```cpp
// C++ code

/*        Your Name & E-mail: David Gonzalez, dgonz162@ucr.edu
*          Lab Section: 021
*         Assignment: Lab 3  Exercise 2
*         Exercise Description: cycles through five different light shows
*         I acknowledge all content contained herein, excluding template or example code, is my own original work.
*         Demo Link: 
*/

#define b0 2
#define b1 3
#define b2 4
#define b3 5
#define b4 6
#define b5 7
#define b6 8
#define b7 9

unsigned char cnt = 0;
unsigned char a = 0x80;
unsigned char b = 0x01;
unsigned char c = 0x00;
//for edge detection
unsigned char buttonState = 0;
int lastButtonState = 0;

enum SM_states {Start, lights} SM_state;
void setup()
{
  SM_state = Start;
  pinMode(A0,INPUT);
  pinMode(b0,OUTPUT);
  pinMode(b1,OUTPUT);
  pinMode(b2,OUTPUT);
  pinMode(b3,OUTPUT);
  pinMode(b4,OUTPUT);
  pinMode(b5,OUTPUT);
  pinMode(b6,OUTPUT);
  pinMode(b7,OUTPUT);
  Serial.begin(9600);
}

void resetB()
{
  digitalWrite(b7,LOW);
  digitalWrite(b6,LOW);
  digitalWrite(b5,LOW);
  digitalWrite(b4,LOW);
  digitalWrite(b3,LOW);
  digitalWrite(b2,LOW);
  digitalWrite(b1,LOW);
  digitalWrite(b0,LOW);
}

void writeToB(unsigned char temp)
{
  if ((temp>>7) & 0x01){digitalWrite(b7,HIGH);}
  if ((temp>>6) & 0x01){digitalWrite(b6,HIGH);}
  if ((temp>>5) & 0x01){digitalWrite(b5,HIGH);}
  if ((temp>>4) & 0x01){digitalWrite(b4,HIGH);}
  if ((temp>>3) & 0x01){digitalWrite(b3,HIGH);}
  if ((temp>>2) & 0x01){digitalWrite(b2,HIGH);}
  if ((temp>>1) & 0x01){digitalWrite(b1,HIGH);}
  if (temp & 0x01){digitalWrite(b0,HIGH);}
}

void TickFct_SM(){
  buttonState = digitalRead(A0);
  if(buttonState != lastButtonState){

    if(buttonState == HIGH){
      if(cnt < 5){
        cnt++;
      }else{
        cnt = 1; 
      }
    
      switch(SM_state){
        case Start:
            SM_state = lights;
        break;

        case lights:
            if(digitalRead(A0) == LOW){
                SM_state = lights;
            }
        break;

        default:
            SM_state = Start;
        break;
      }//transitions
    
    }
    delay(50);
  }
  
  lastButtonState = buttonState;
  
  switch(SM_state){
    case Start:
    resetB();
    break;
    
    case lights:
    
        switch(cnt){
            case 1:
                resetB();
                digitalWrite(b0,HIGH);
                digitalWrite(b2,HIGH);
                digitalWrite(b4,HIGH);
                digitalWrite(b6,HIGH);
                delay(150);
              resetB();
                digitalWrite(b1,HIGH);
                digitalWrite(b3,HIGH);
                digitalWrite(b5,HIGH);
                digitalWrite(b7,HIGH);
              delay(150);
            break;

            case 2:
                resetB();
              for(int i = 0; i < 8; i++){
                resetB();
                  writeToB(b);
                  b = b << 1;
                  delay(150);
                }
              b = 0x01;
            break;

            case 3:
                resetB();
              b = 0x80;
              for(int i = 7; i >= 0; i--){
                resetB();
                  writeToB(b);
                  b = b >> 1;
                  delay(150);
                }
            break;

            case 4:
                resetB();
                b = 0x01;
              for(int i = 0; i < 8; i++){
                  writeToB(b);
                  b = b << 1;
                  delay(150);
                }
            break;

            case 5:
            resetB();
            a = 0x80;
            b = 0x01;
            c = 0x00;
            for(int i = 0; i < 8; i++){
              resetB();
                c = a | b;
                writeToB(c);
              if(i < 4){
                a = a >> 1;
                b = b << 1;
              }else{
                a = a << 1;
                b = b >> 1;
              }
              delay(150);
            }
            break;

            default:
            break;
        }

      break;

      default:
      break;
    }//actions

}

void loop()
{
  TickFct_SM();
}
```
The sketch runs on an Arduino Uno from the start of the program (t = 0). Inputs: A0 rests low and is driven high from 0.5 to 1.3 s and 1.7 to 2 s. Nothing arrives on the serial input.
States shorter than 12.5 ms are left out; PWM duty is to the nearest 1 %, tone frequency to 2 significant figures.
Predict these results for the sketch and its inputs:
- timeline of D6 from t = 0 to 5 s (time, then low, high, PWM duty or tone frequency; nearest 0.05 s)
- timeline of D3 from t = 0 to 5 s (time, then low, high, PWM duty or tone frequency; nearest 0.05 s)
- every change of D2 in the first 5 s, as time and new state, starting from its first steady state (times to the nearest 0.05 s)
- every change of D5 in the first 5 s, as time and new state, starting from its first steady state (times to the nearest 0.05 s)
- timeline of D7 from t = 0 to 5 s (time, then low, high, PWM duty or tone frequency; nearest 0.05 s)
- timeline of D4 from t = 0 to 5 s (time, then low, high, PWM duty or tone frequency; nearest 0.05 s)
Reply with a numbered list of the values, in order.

1. 0 s low; 0.55 s high; 0.7 s low; 0.85 s high; 1 s low; 1.15 s high; 1.3 s low; 1.5 s high; 1.65 s low; 2.45 s high; 2.6 s low; 3.7 s high; 3.85 s low; 4.9 s high
2. 0 s low; 0.7 s high; 0.85 s low; 1 s high; 1.15 s low; 1.3 s high; 1.5 s low; 1.65 s high; 1.85 s low; 2 s high; 2.15 s low; 3.25 s high; 3.4 s low; 4.45 s high; 4.6 s low
3. 0 s low; 0.55 s high; 0.7 s low; 0.85 s high; 1 s low; 1.15 s high; 1.3 s low; 1.5 s high; 1.65 s low; 1.85 s high; 2 s low; 3.1 s high; 3.25 s low; 4.3 s high; 4.45 s low
4. 0 s low; 0.7 s high; 0.85 s low; 1 s high; 1.15 s low; 1.3 s high; 1.5 s low; 1.65 s high; 1.85 s low; 2.3 s high; 2.45 s low; 3.55 s high; 3.7 s low; 4.75 s high; 4.9 s low
5. 0 s low; 0.7 s high; 0.85 s low; 1 s high; 1.15 s low; 1.3 s high; 1.5 s low; 1.65 s high; 1.85 s low; 2.6 s high; 2.75 s low; 3.85 s high; 4 s low
6. 0 s low; 0.55 s high; 0.7 s low; 0.85 s high; 1 s low; 1.15 s high; 1.3 s low; 1.5 s high; 1.65 s low; 2.15 s high; 2.3 s low; 3.4 s high; 3.55 s low; 4.6 s high; 4.75 s low
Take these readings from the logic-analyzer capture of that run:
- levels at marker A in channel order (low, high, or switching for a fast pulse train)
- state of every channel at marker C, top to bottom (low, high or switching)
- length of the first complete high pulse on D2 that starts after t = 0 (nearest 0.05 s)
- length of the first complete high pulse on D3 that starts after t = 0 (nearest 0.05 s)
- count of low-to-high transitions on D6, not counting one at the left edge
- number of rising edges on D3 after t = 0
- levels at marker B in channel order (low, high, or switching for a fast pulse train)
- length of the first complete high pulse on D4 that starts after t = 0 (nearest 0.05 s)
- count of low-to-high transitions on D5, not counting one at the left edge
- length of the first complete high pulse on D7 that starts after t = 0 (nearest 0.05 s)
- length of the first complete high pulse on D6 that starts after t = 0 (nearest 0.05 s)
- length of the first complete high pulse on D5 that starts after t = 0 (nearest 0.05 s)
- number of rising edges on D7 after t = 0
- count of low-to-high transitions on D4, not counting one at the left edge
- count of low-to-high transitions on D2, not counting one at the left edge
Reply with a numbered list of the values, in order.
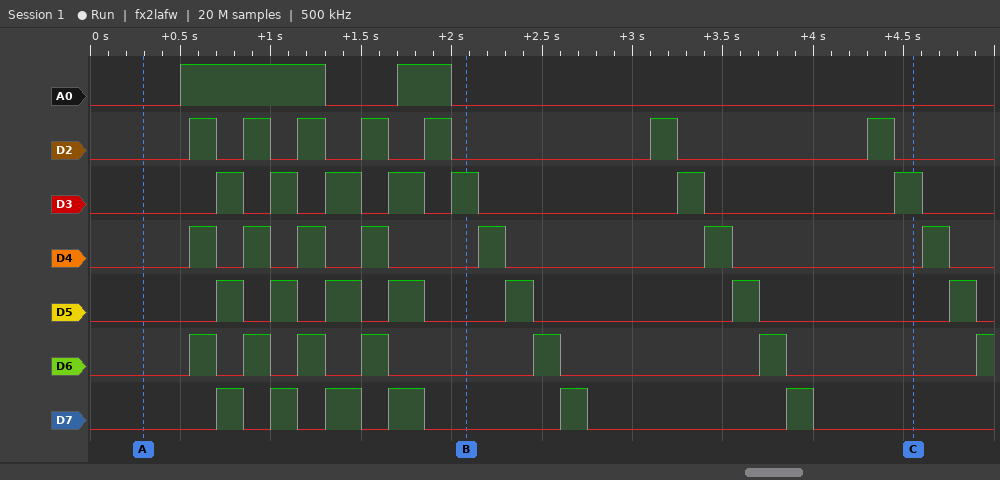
1. A0 low, D2 low, D3 low, D4 low, D5 low, D6 low, D7 low
2. A0 low, D2 low, D3 high, D4 low, D5 low, D6 low, D7 low
3. 0.15 s
4. 0.15 s
5. 7
6. 7
7. A0 low, D2 low, D3 high, D4 low, D5 low, D6 low, D7 low
8. 0.15 s
9. 7
10. 0.15 s
11. 0.15 s
12. 0.15 s
13. 6
14. 7
15. 7
